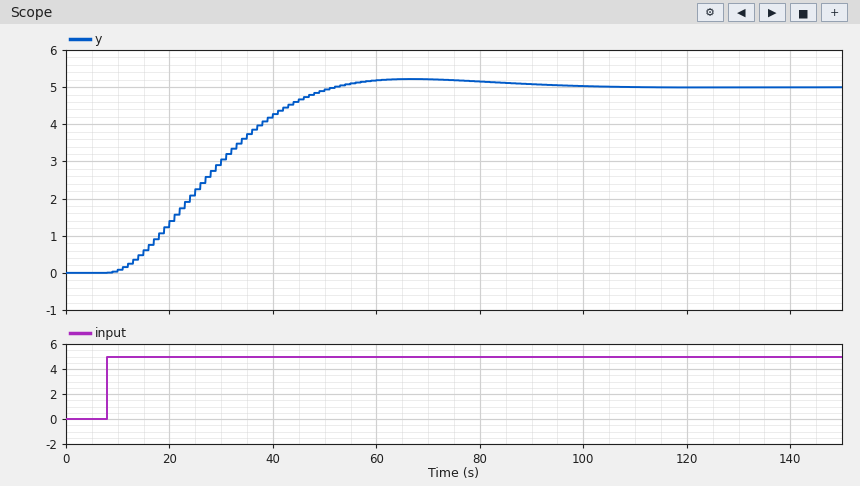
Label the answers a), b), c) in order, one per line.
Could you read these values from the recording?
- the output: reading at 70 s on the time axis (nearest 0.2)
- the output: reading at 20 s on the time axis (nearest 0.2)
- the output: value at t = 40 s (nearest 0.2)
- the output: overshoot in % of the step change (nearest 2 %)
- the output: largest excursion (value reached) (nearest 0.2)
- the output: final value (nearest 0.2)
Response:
a) 5.2
b) 1.4
c) 4.2
d) 4 %
e) 5.2
f) 5.0
